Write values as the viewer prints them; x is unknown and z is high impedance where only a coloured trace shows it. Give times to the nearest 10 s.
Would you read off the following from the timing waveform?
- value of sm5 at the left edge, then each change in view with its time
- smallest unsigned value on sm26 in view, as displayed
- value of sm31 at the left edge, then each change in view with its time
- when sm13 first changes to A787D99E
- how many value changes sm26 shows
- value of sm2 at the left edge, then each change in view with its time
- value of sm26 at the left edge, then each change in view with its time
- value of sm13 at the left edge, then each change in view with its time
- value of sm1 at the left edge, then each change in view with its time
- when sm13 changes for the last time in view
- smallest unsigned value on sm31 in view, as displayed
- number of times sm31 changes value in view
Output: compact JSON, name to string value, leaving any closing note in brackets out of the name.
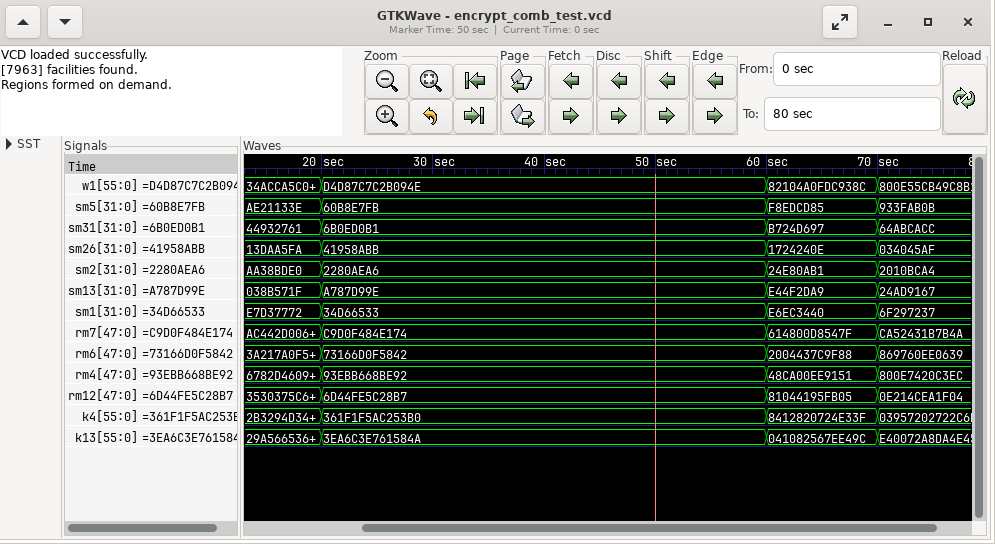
{"value of sm5 at the left edge, then each change in view with its time": "AE21133E, 60B8E7FB at 20 s, F8EDCD85 at 60 s, 933FAB0B at 70 s", "smallest unsigned value on sm26 in view, as displayed": "034045AF", "value of sm31 at the left edge, then each change in view with its time": "44932761, 6B0ED0B1 at 20 s, B724D697 at 60 s, 64ABCACC at 70 s", "when sm13 first changes to A787D99E": "20 s", "how many value changes sm26 shows": "3", "value of sm2 at the left edge, then each change in view with its time": "AA38BDE0, 2280AEA6 at 20 s, 24E80AB1 at 60 s, 2010BCA4 at 70 s", "value of sm26 at the left edge, then each change in view with its time": "13DAA5FA, 41958ABB at 20 s, 1724240E at 60 s, 034045AF at 70 s", "value of sm13 at the left edge, then each change in view with its time": "038B571F, A787D99E at 20 s, E44F2DA9 at 60 s, 24AD9167 at 70 s", "value of sm1 at the left edge, then each change in view with its time": "E7D37772, 34D66533 at 20 s, E6EC3440 at 60 s, 6F297237 at 70 s", "when sm13 changes for the last time in view": "70 s", "smallest unsigned value on sm31 in view, as displayed": "44932761", "number of times sm31 changes value in view": "3"}
